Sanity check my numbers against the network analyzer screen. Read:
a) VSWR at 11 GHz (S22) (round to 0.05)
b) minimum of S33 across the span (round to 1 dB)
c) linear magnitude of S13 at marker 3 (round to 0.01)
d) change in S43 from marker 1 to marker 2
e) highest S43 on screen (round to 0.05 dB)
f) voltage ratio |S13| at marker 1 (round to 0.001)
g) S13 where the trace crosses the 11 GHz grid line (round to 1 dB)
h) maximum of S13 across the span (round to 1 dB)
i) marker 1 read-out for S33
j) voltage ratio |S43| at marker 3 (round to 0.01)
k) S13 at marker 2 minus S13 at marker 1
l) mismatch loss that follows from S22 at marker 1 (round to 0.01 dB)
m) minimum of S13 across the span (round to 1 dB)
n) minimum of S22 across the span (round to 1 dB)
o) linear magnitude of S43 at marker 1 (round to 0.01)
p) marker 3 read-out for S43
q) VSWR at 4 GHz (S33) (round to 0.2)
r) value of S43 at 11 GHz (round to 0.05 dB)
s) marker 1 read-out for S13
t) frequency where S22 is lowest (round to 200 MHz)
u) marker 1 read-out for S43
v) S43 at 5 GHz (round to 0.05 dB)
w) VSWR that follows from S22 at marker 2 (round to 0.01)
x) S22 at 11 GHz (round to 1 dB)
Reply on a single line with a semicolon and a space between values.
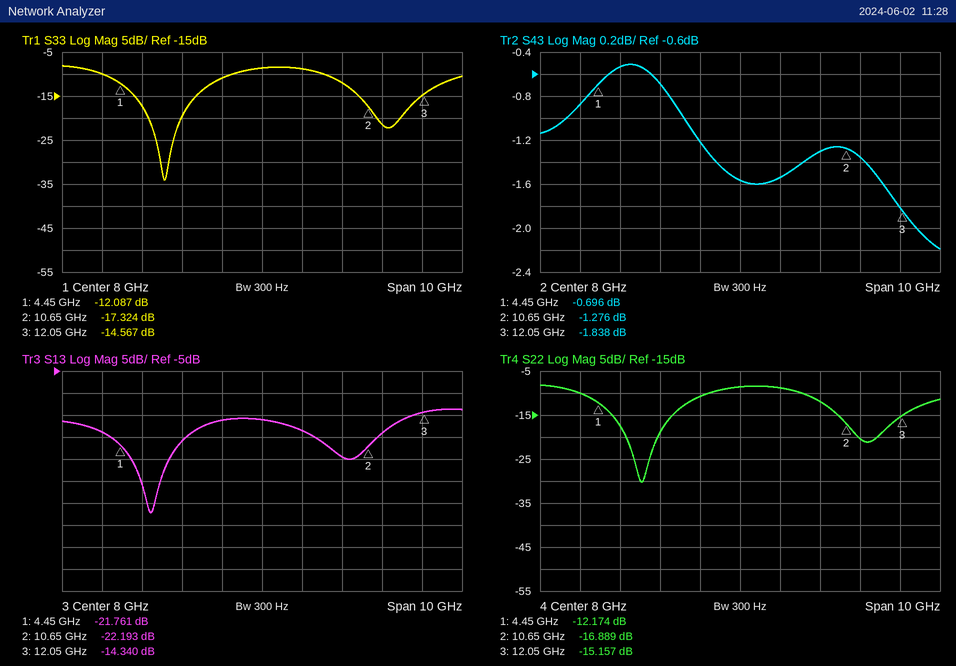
1.20; -34 dB; 0.19; -0.580 dB; -0.50 dB; 0.082; -19 dB; -14 dB; -12.087 dB; 0.81; -0.432 dB; 0.27 dB; -37 dB; -30 dB; 0.92; -1.838 dB; 2.0; -1.35 dB; -21.761 dB; 5.6 GHz; -0.696 dB; -0.55 dB; 1.33; -20 dB
